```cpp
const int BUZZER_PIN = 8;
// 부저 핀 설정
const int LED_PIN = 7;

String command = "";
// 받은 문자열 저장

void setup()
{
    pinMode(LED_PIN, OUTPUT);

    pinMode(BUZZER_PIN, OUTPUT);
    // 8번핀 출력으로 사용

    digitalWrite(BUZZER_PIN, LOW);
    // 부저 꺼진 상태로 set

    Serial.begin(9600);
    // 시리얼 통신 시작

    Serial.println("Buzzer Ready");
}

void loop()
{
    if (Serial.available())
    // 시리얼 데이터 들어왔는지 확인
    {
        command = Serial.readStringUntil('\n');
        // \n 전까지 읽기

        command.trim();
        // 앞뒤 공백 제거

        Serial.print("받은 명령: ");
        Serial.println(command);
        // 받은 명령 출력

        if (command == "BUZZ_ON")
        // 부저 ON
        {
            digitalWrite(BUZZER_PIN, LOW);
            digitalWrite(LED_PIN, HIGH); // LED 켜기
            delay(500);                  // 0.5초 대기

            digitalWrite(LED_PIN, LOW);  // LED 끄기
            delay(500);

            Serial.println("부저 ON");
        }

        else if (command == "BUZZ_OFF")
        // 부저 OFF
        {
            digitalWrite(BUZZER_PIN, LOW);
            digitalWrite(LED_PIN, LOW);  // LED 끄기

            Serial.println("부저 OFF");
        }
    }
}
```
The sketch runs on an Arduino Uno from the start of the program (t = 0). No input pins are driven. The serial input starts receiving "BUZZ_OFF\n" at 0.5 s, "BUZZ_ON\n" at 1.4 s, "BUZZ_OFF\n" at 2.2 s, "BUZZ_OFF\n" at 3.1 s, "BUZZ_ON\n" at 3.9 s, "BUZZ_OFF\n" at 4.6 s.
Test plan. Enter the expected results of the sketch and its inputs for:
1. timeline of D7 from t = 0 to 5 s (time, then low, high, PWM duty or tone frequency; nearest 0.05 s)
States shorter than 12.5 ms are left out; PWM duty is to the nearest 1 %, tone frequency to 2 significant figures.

0 s low; 1.4 s high; 1.9 s low; 3.9 s high; 4.4 s low
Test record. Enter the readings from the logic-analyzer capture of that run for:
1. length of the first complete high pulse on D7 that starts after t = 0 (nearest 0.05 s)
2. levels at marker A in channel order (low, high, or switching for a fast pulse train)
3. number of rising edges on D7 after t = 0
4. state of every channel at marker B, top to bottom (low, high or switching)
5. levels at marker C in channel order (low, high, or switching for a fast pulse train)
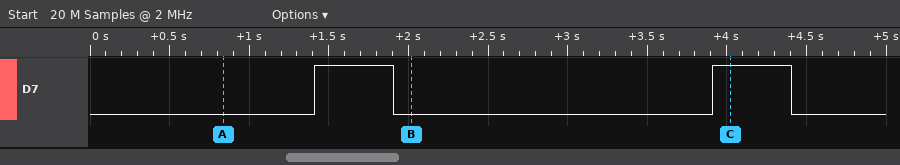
0.50 s
D7 low
2
D7 low
D7 high
